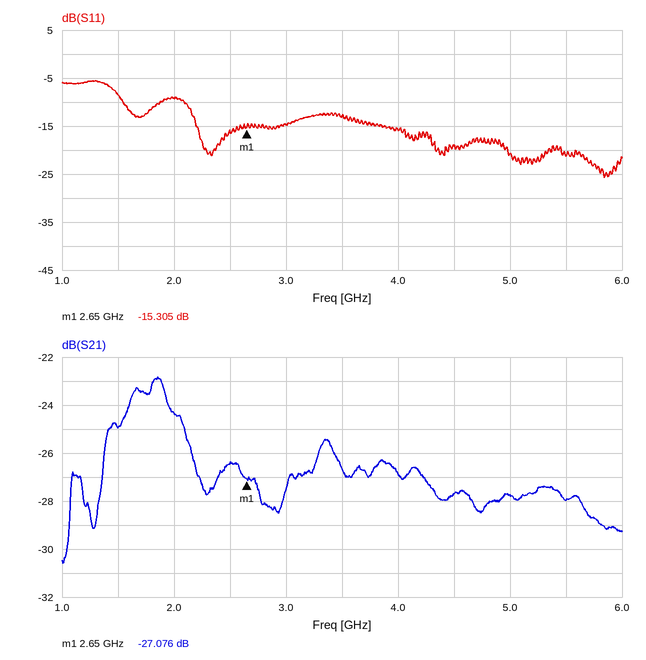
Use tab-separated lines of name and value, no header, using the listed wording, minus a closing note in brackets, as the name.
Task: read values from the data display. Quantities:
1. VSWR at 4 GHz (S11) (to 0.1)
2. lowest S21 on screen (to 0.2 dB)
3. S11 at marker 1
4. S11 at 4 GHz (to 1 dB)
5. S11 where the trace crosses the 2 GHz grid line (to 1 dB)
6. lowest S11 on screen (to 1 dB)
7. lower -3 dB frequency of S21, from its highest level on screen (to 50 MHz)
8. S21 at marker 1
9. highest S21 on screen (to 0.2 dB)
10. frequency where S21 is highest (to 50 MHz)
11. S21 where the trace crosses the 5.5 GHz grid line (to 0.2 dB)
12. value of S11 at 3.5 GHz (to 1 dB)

VSWR at 4 GHz (S11)	1.4
lowest S21 on screen	-30.6 dB
S11 at marker 1	-15.305 dB
S11 at 4 GHz	-16 dB
S11 where the trace crosses the 2 GHz grid line	-9 dB
lowest S11 on screen	-26 dB
lower -3 dB frequency of S21, from its highest level on screen	1.40 GHz
S21 at marker 1	-27.076 dB
highest S21 on screen	-22.8 dB
frequency where S21 is highest	1.85 GHz
S21 where the trace crosses the 5.5 GHz grid line	-28.0 dB
value of S11 at 3.5 GHz	-13 dB
